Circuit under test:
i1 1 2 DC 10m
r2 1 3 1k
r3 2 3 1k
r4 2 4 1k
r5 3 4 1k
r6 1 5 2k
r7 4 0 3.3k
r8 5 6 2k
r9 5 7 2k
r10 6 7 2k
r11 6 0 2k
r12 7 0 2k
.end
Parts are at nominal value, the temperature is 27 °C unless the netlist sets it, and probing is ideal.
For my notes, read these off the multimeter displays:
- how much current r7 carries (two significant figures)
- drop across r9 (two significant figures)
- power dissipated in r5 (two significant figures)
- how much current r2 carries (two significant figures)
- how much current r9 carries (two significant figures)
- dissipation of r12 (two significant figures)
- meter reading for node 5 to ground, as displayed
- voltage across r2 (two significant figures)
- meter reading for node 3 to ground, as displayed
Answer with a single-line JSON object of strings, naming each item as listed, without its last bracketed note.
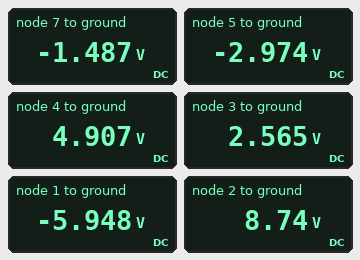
{"how much current r7 carries": "1.5 mA", "drop across r9": "1.5 V", "power dissipated in r5": "5.5 mW", "how much current r2 carries": "8.5 mA", "how much current r9 carries": "740 µA", "dissipation of r12": "1.1 mW", "meter reading for node 5 to ground, as displayed": "-2.974 V", "voltage across r2": "8.5 V", "meter reading for node 3 to ground, as displayed": "2.565 V"}
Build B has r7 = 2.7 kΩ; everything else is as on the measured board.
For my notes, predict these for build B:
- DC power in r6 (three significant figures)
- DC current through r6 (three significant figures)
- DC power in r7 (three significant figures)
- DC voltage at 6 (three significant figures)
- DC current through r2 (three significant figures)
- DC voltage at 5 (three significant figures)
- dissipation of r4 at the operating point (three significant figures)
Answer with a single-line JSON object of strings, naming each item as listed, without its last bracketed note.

{"DC power in r6": "5.08 mW", "DC current through r6": "1.59 mA", "DC power in r7": "6.86 mW", "DC voltage at 6": "-1.59 V", "DC current through r2": "8.41 mA", "DC voltage at 5": "-3.19 V", "dissipation of r4 at the operating point": "14.9 mW"}
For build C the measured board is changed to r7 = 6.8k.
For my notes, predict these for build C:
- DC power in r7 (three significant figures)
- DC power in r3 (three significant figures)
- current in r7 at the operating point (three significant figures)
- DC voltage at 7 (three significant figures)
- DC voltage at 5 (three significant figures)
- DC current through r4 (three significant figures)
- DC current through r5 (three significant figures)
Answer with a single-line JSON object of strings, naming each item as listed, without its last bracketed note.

{"DC power in r7": "7.78 mW", "DC power in r3": "39.8 mW", "current in r7 at the operating point": "1.07 mA", "DC voltage at 7": "-1.07 V", "DC voltage at 5": "-2.14 V", "DC current through r4": "3.69 mA", "DC current through r5": "2.62 mA"}
